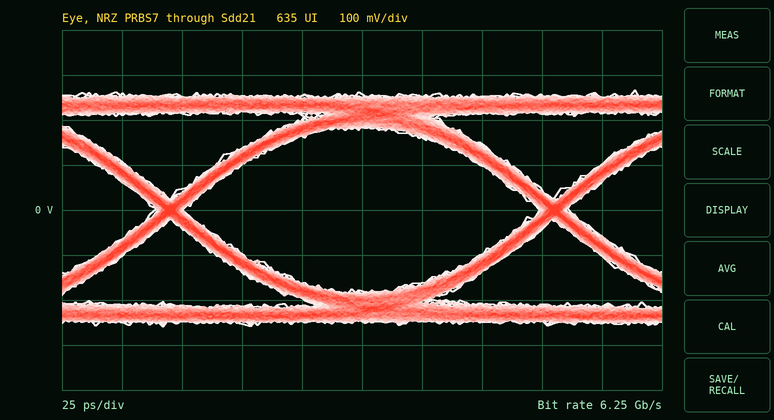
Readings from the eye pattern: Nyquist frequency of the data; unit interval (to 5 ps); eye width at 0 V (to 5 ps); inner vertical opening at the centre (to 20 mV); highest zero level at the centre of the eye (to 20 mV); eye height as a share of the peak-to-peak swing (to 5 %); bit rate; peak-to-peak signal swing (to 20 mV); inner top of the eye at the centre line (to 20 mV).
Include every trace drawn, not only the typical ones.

3.125 GHz
160 ps
150 ps
360 mV
-180 mV
70 %
6.25 Gb/s
520 mV
180 mV
